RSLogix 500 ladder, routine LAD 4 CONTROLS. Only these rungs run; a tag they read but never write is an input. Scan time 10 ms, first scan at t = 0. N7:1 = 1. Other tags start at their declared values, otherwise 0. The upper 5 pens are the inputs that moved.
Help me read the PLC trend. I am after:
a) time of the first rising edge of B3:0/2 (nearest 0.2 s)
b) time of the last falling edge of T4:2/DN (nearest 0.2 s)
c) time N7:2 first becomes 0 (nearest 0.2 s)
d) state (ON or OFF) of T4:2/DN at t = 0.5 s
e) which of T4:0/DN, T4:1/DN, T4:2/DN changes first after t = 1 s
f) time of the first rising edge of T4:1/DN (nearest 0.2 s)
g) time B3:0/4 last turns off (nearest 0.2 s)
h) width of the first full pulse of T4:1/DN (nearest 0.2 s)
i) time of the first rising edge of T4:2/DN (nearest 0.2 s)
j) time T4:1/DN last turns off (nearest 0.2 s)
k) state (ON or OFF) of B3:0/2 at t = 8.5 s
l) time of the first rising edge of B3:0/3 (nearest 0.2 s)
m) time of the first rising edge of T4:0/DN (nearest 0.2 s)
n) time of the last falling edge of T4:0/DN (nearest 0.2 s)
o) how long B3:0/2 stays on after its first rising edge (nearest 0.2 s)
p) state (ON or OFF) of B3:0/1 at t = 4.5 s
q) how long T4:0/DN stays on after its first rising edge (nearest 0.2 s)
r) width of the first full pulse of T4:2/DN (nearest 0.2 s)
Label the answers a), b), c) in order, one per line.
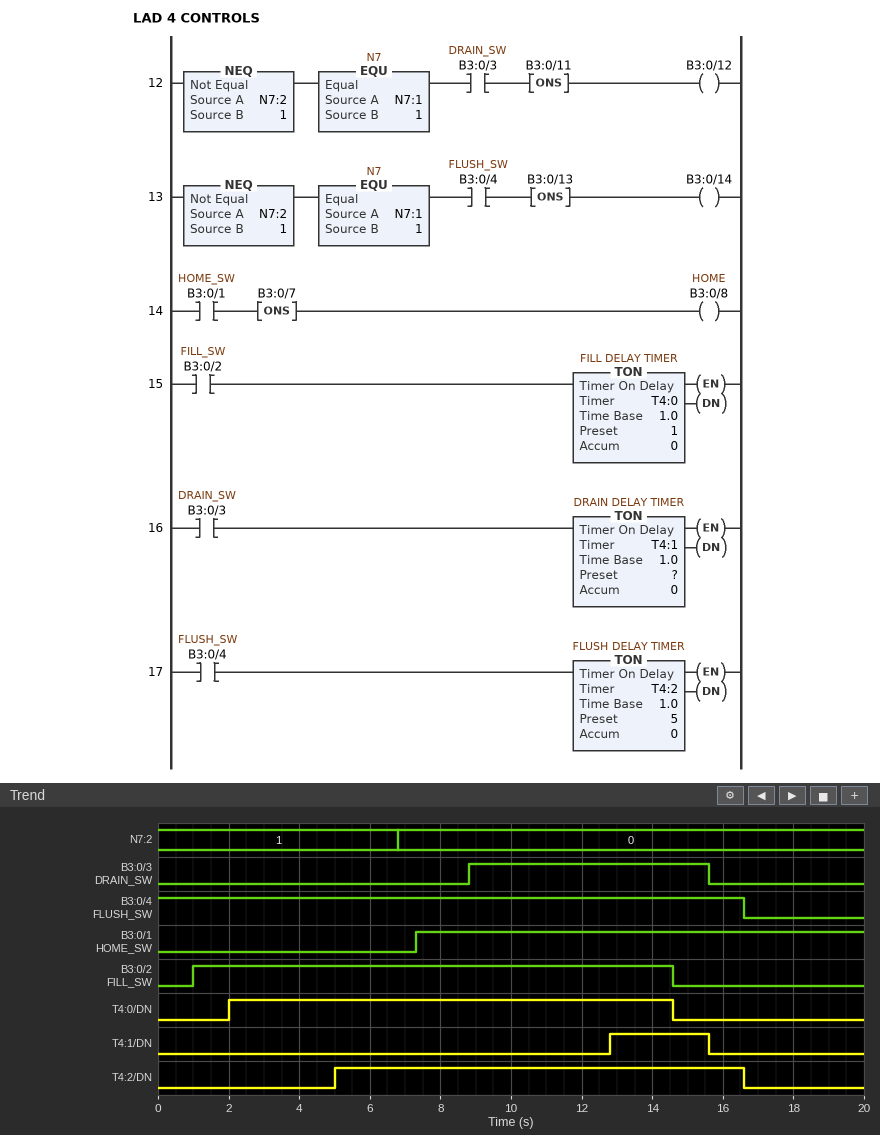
a) 1.0 s
b) 16.6 s
c) 6.8 s
d) OFF
e) T4:0/DN
f) 12.8 s
g) 16.6 s
h) 2.8 s
i) 5.0 s
j) 15.6 s
k) ON
l) 8.8 s
m) 2.0 s
n) 14.6 s
o) 13.6 s
p) OFF
q) 12.6 s
r) 11.6 s
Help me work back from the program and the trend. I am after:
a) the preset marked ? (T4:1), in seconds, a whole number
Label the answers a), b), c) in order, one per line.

a) 4 s
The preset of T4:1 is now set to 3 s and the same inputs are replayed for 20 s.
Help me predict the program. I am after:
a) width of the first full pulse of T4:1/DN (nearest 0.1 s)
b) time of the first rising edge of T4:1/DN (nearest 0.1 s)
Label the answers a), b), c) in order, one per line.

a) 3.8 s
b) 11.8 s
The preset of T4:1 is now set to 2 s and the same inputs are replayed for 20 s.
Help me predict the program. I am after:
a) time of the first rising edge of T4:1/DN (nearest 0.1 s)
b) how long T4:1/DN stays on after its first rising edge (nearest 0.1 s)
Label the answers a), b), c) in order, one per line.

a) 10.8 s
b) 4.8 s
